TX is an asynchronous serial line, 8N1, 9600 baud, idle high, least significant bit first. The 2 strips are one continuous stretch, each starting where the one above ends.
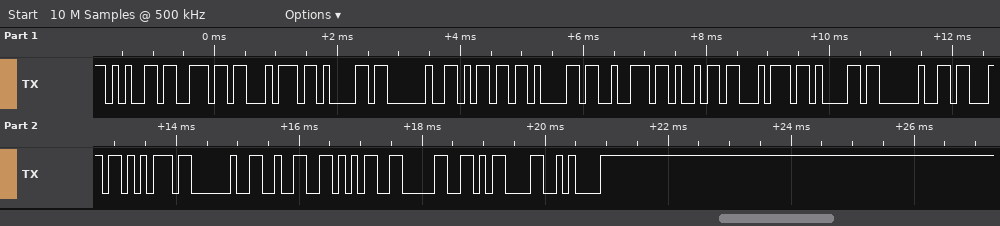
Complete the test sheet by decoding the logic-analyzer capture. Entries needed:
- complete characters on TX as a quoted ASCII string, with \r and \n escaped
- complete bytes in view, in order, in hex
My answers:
"enta marita cu 250\r\n"
65 6E 74 61 20 6D 61 72 69 74 61 20 63 75 20 32 35 30 0D 0A
